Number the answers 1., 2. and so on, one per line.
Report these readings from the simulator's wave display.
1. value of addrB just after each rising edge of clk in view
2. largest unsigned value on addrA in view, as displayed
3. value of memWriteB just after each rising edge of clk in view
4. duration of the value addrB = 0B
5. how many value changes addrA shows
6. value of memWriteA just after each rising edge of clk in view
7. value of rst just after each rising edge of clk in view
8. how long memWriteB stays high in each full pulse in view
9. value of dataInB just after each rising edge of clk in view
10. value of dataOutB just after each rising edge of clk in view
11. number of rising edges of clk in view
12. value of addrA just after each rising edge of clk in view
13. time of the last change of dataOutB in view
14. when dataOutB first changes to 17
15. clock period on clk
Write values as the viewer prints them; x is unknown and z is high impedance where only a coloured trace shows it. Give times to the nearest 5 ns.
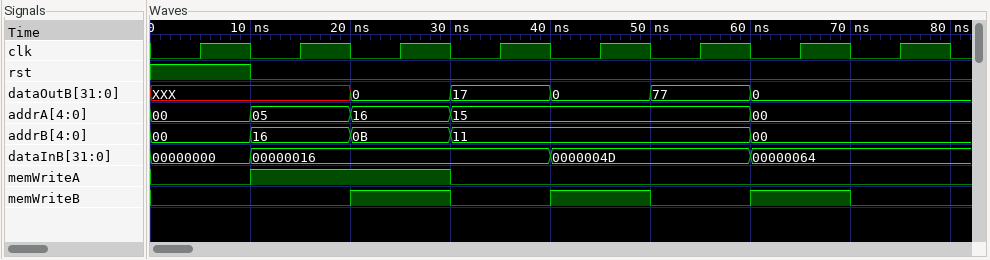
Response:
1. 00, 16, 0B, 11, 11, 11, 00, 00
2. 16
3. 0 0 1 0 1 0 1 0
4. 10 ns
5. 4
6. 0 1 1 0 0 0 0 0
7. 1 0 0 0 0 0 0 0
8. 10 ns, 10 ns, 10 ns
9. 00000000, 00000016, 00000016, 00000016, 0000004D, 0000004D, 00000064, 00000064
10. XXX, XXX, 0, 17, 0, 77, 0, 0
11. 8
12. 00, 05, 16, 15, 15, 15, 00, 00
13. 60 ns
14. 30 ns
15. 10 ns
